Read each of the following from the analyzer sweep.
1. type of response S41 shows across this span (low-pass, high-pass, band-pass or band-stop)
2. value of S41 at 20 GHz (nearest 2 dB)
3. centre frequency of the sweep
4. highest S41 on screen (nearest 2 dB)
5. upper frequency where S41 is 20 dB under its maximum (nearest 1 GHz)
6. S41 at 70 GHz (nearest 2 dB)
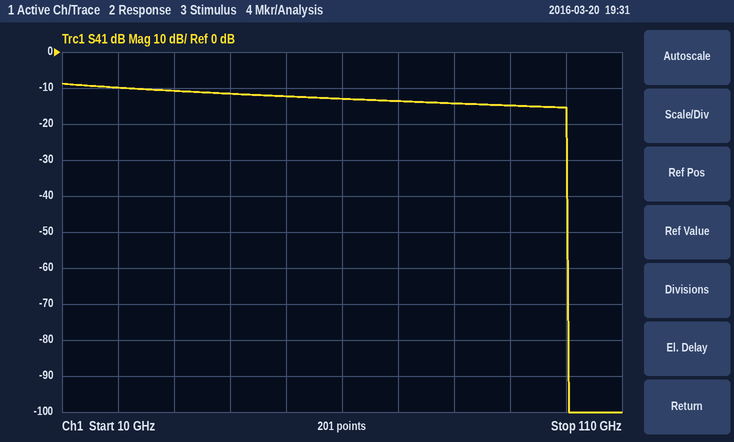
low-pass
-10 dB
60 GHz
-8 dB
100 GHz
-14 dB
